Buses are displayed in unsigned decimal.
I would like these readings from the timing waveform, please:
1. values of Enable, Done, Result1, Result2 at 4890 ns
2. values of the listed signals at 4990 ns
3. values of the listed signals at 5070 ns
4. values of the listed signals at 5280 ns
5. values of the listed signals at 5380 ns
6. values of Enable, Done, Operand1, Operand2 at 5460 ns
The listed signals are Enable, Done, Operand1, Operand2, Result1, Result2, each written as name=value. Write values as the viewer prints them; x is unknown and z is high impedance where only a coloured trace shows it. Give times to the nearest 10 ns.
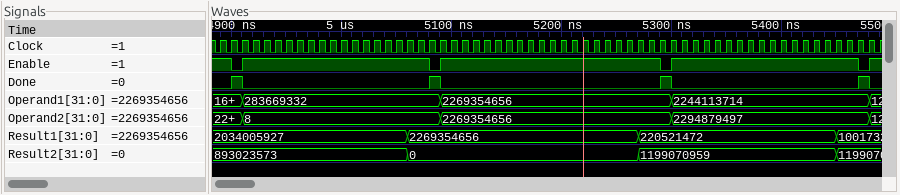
Enable=1, Done=0, Result1=2034005927, Result2=893023573
Enable=1, Done=0, Operand1=283669332, Operand2=8, Result1=2034005927, Result2=893023573
Enable=1, Done=0, Operand1=283669332, Operand2=8, Result1=2269354656, Result2=0
Enable=1, Done=0, Operand1=2269354656, Operand2=2269354656, Result1=220521472, Result2=1199070959
Enable=1, Done=0, Operand1=2244113714, Operand2=2294879497, Result1=220521472, Result2=1199070959
Enable=1, Done=0, Operand1=2244113714, Operand2=2294879497
